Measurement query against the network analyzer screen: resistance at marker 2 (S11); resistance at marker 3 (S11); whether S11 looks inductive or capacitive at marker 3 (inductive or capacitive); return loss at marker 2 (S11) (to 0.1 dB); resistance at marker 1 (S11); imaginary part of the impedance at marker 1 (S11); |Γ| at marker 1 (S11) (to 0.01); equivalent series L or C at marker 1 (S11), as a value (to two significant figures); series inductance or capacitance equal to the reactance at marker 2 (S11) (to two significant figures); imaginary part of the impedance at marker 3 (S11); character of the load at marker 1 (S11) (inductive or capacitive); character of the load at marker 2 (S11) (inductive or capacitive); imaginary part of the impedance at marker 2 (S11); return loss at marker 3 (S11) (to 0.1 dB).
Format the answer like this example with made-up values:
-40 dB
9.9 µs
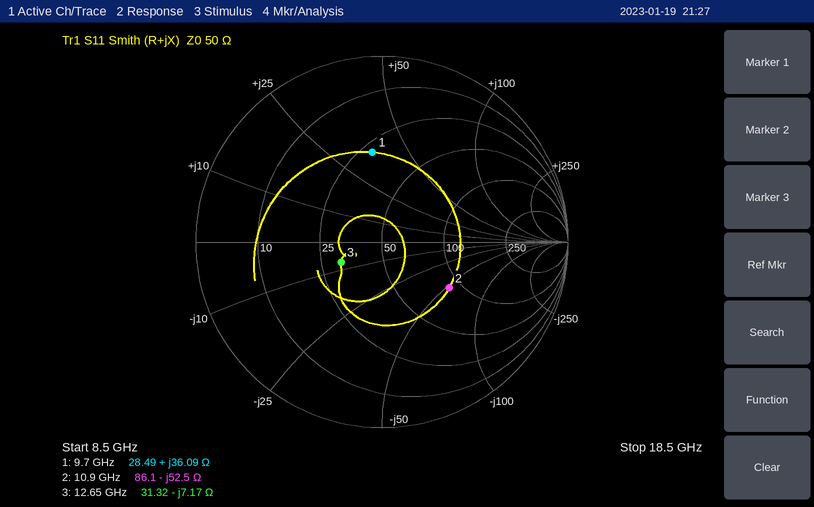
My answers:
86.1 Ω
31.32 Ω
capacitive
7.2 dB
28.49 Ω
+36.09 Ω
0.49
590 pH
280 fF
-7.17 Ω
inductive
capacitive
-52.5 Ω
12.2 dB
